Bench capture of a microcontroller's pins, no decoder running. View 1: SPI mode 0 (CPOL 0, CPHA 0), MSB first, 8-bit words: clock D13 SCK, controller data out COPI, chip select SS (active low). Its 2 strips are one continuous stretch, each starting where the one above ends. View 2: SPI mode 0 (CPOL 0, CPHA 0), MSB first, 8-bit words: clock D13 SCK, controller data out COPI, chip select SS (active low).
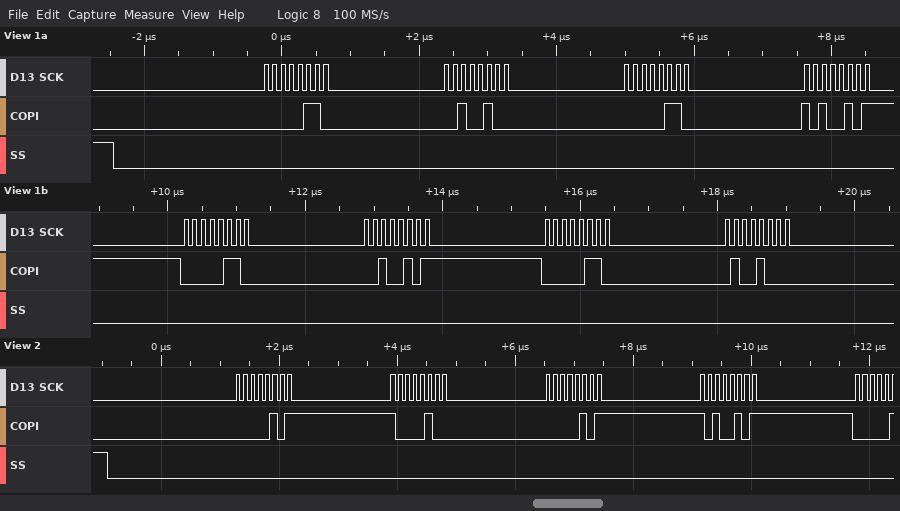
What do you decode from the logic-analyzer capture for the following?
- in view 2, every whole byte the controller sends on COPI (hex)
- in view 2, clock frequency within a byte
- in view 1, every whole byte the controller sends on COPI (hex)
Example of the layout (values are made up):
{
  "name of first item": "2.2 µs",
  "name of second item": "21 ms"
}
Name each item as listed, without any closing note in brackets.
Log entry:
{
  "in view 2, every whole byte the controller sends on COPI": "05 84 05 A5",
  "in view 2, clock frequency within a byte": "8 MHz",
  "in view 1, every whole byte the controller sends on COPI": "06 24 06 A5 06 25 06 48"
}
